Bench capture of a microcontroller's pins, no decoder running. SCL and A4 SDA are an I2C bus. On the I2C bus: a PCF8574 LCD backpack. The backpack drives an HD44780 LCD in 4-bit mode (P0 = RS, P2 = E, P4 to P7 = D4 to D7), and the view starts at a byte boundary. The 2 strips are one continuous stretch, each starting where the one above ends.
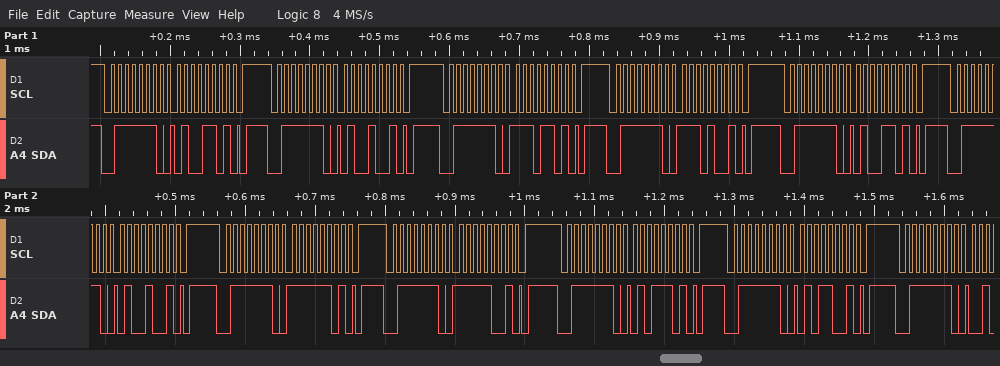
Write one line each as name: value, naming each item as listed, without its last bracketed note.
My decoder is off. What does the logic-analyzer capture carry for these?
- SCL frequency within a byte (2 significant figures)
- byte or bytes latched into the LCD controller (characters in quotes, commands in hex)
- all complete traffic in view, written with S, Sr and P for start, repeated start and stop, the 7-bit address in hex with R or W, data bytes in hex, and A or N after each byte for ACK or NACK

SCL frequency within a byte: 100 kHz
byte or bytes latched into the LCD controller: 'N' 'O'
all complete traffic in view, written with S, Sr and P for start, repeated start and stop, the 7-bit address in hex with R or W, data bytes in hex, and A or N after each byte for ACK or NACK: S 3FW A 4D A P S 3FW A 49 A P S 3FW A ED A P S 3FW A E9 A P S 3FW A 4D A P S 3FW A 49 A P S 3FW A FD A P S 3FW A F9 A P S 3FW A 5D A P S 3FW A 59 A P S 3FW A
